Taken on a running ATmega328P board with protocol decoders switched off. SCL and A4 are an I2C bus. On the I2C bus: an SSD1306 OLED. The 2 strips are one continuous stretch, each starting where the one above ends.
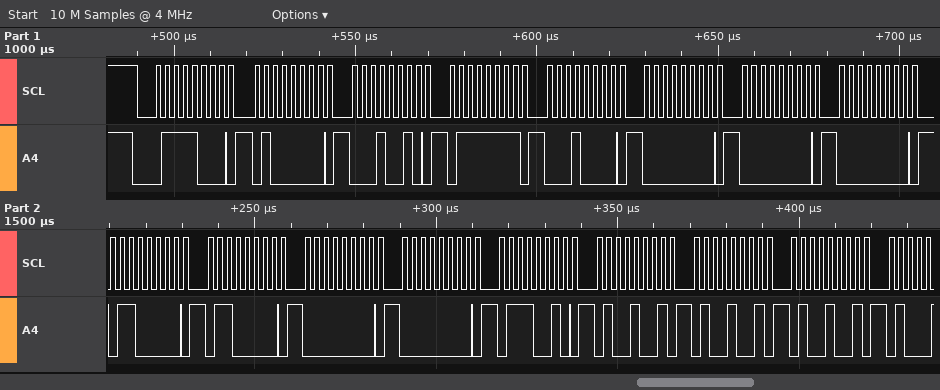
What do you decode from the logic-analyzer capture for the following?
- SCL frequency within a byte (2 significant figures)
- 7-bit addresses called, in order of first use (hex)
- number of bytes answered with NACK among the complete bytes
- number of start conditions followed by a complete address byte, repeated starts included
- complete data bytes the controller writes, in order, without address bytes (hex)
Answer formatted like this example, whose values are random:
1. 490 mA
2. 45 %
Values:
1. 400 kHz
2. 0x3C
3. 0
4. 1
5. 40 12 7F 10 00 00 00 60 60 00 00 72 49 49 49
